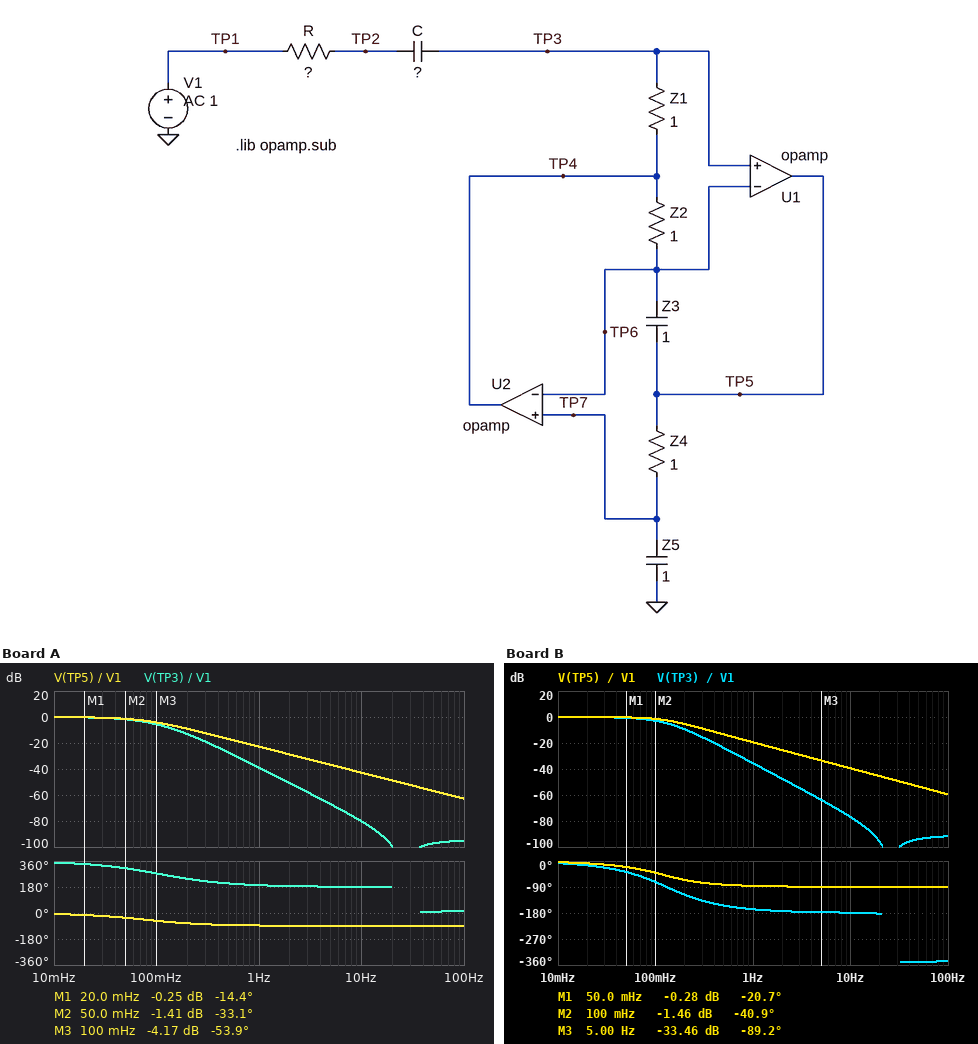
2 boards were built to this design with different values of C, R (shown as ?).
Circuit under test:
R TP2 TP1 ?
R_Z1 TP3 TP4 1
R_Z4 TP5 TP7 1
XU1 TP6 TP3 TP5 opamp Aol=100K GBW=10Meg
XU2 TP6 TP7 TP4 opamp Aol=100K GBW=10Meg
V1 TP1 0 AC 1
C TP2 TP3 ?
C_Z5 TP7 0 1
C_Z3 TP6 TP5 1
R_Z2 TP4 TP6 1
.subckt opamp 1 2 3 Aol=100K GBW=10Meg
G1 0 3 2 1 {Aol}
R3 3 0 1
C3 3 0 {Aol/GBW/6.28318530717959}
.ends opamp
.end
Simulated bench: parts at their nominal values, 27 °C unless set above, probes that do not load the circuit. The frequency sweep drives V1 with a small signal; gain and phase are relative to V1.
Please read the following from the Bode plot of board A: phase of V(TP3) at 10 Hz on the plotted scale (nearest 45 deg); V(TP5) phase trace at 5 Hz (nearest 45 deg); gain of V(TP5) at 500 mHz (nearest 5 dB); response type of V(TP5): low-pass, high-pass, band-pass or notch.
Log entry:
180 deg
-90 deg
-15 dB
low-pass
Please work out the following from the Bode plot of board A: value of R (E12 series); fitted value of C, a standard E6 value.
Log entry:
2.2 Ω
330 mF
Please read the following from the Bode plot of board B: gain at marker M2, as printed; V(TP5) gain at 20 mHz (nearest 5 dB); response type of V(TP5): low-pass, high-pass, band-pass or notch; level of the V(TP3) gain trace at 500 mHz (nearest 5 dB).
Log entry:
-1.46 dB
0 dB
low-pass
-25 dB
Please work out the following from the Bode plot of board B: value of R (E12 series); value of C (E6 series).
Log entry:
1.5 Ω
470 mF
